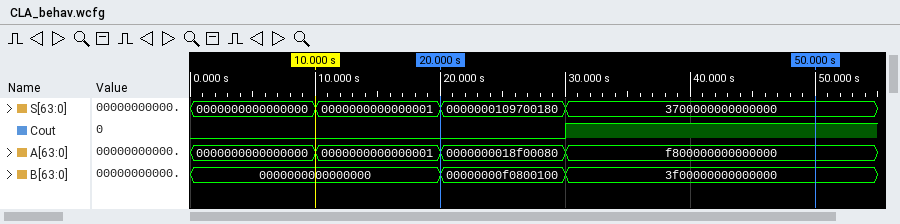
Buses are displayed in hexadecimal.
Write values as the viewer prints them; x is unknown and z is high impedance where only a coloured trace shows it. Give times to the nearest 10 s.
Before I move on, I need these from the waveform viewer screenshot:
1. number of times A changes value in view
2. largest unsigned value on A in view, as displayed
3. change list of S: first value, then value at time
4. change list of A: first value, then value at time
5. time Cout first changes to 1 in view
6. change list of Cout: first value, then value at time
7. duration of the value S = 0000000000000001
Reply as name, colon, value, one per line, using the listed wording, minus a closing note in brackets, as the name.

number of times A changes value in view: 3
largest unsigned value on A in view, as displayed: f800000000000000
change list of S: first value, then value at time: 0000000000000000, 0000000000000001 at 10 s, 0000000109700180 at 20 s, 3700000000000000 at 30 s
change list of A: first value, then value at time: 0000000000000000, 0000000000000001 at 10 s, 0000000018f00080 at 20 s, f800000000000000 at 30 s
time Cout first changes to 1 in view: 30 s
change list of Cout: first value, then value at time: 0, 1 at 30 s
duration of the value S = 0000000000000001: 10 s
